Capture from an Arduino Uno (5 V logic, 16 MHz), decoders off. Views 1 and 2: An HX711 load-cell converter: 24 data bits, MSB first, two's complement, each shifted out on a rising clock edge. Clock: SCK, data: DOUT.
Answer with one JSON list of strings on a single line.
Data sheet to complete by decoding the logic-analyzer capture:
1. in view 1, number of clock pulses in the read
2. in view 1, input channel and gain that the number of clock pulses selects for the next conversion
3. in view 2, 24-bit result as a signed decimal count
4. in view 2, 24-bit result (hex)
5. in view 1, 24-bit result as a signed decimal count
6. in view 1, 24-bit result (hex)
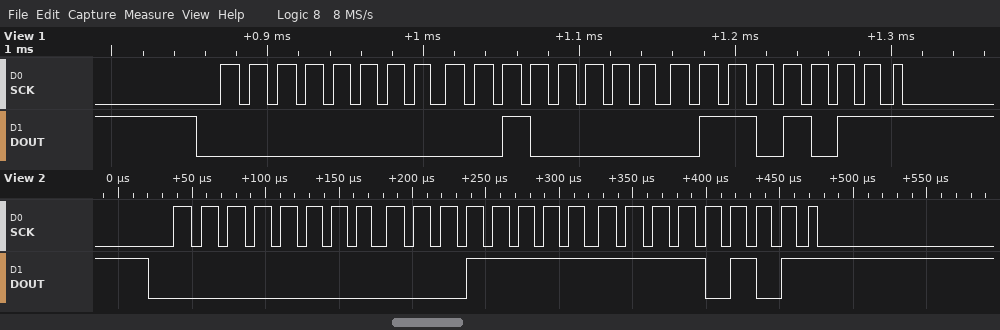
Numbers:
["25", "channel A, gain 128", "8181", "0x001FF5", "8299", "0x00206B"]
